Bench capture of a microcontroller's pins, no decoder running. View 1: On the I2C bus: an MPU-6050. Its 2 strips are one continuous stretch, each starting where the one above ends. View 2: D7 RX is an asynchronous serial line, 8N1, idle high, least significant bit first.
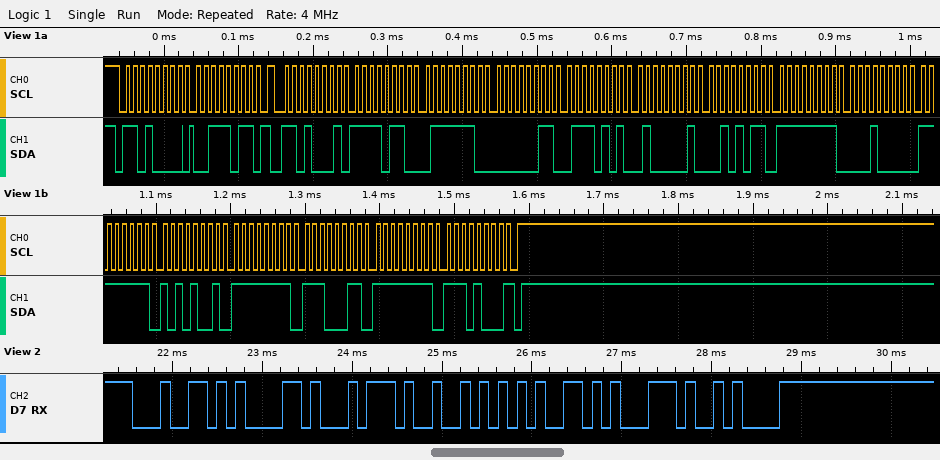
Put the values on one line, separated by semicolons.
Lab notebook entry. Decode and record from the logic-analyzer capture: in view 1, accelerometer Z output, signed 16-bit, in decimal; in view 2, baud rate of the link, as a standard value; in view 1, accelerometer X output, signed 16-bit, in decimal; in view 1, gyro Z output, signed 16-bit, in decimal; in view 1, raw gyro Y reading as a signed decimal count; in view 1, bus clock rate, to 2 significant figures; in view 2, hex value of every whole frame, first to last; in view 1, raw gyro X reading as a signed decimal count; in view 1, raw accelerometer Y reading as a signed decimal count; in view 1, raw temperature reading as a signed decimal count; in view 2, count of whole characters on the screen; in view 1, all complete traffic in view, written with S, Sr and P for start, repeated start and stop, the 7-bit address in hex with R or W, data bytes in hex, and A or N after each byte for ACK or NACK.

16683; 9600 baud; -2434; -24; -29; 100 kHz; 0x64 0x61 0x74 0x52 0x65 0x71 0x0A; -87; 885; -240; 7; S 68W A 3B A Sr 68R A F6 A 7E A 03 A 75 A 41 A 2B A FF A 10 A FF A A9 A FF A E3 A FF A E8 N P
